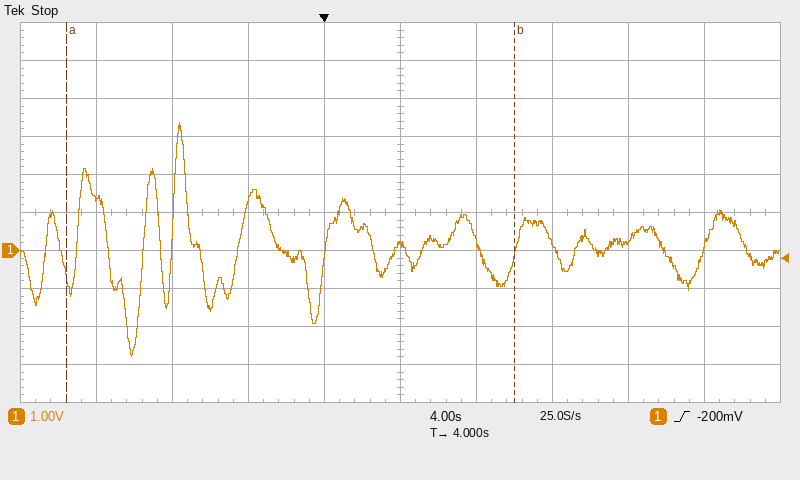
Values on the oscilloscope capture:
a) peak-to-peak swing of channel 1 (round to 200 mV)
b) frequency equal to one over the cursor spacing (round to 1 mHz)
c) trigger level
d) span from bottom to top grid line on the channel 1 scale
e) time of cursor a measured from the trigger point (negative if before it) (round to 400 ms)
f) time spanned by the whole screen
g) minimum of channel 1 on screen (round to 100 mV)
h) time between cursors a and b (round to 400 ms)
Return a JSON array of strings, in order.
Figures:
["6.2 V", "42 mHz", "-200 mV", "10 V", "-13.6 s", "40 s", "-2.8 V", "23.6 s"]
